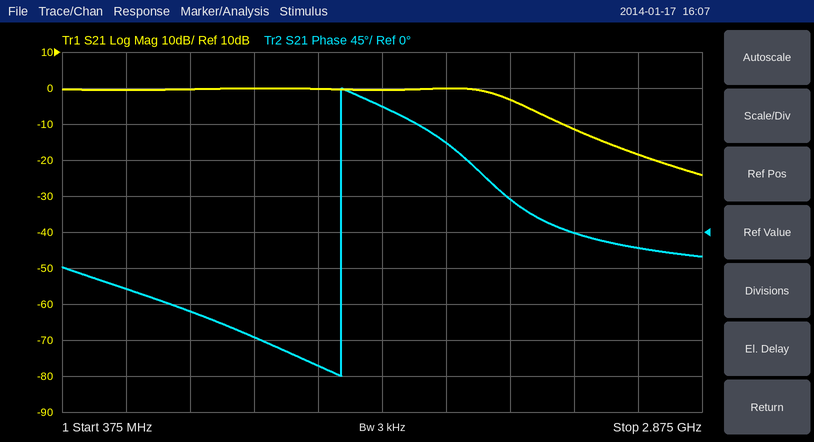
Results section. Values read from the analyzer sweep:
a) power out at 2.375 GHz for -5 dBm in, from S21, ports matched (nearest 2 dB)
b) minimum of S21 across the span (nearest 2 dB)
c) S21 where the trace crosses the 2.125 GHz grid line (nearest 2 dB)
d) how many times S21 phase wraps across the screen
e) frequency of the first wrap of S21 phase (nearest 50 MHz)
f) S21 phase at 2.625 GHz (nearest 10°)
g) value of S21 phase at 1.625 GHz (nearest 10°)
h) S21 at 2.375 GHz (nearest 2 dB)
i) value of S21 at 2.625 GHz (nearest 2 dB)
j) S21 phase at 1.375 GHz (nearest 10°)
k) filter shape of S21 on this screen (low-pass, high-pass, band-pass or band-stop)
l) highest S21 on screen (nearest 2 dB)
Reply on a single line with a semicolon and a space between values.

-16 dBm; -24 dB; -4 dB; 1; 1.45 GHz; -20°; 160°; -12 dB; -18 dB; -170°; low-pass; 0 dB
